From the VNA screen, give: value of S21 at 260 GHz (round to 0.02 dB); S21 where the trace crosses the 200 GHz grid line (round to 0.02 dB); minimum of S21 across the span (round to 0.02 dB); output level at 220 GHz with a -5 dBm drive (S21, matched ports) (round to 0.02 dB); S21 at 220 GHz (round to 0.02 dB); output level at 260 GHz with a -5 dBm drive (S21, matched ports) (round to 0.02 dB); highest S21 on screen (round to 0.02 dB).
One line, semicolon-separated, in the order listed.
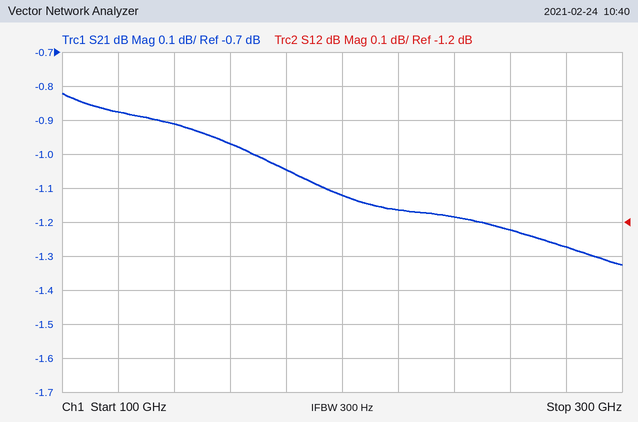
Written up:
-1.22 dB; -1.12 dB; -1.32 dB; -6.16 dBm; -1.16 dB; -6.22 dBm; -0.82 dB
